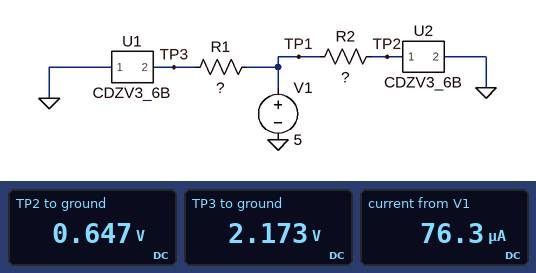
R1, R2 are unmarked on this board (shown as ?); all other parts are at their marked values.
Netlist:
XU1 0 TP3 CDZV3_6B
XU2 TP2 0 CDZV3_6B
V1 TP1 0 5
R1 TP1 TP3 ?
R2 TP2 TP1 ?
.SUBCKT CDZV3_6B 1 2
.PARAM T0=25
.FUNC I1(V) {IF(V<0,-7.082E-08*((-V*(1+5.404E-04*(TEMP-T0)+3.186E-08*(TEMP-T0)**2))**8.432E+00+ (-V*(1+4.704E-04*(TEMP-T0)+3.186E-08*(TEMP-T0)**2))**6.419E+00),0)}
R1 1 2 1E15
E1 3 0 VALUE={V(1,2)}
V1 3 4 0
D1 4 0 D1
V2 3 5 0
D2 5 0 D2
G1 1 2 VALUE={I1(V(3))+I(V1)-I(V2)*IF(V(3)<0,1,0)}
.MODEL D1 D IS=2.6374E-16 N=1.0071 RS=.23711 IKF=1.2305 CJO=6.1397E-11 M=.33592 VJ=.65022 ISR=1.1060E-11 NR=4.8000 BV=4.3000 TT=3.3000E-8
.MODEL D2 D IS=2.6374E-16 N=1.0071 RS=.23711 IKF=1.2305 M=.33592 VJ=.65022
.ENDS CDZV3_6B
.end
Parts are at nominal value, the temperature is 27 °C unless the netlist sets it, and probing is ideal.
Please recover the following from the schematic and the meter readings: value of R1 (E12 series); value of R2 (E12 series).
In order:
47 kΩ
270 kΩ
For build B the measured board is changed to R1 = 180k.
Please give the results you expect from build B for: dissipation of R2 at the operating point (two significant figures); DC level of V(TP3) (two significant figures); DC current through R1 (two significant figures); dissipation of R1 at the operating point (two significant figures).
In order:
70 µW
1.9 V
17 µA
55 µW
